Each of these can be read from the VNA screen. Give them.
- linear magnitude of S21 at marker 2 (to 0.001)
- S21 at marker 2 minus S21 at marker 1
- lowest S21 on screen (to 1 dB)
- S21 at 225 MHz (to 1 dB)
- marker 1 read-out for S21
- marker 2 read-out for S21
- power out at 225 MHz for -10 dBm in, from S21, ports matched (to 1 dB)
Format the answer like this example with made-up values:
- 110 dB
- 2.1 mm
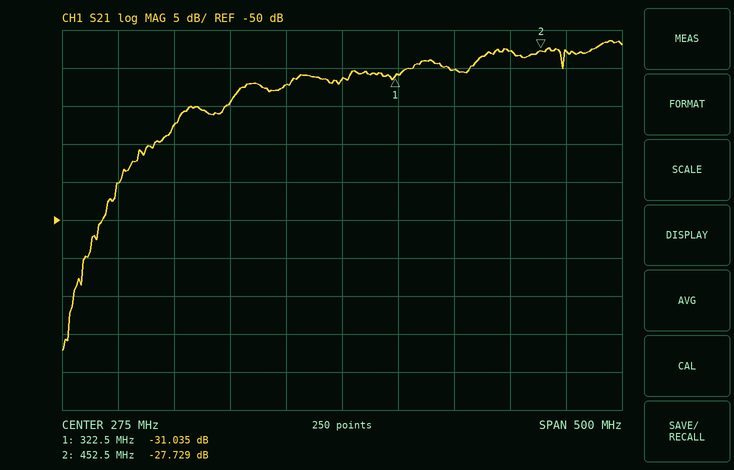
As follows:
- 0.041
- 3.306 dB
- -67 dB
- -32 dB
- -31.035 dB
- -27.729 dB
- -42 dBm
